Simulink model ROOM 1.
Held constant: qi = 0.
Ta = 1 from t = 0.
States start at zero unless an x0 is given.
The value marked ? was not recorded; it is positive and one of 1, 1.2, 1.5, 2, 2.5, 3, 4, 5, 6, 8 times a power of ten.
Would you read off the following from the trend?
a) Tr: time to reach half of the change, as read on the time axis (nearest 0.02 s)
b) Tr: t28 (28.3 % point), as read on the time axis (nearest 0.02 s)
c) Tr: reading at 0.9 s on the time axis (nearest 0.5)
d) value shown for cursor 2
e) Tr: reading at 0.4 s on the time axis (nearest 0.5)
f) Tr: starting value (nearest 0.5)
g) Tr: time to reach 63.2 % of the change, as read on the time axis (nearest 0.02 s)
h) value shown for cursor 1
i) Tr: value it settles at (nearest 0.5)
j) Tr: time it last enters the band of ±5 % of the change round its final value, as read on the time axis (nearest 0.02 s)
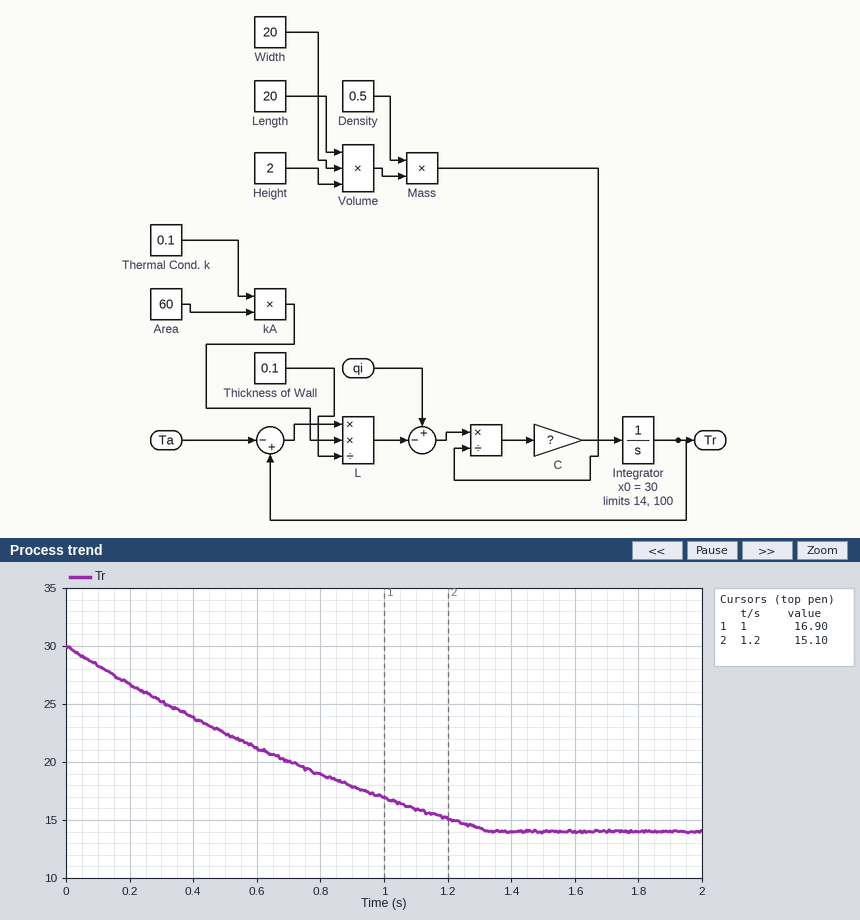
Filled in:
0.54 s
0.28 s
18.0
15.10
24.0
30.0
0.72 s
16.90
14.0
1.24 s
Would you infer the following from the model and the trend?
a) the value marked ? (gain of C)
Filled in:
4
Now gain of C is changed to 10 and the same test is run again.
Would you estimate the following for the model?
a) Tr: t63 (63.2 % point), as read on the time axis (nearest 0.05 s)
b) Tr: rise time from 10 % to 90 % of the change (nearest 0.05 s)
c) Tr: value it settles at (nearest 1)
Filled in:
0.30 s
0.40 s
14
